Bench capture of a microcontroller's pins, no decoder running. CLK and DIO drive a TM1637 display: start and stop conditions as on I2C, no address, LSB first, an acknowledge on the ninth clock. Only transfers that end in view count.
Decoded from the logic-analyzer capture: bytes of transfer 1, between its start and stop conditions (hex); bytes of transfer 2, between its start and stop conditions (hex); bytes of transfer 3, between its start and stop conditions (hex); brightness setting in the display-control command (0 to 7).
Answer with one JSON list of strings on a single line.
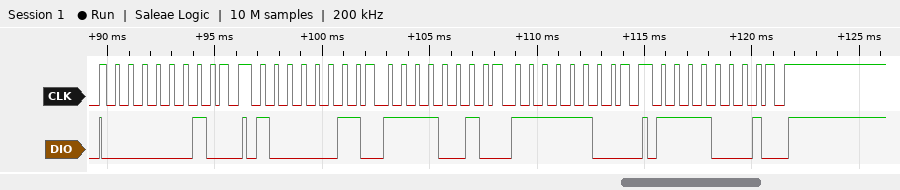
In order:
["40", "C1 4F 3F", "8F", "7"]
